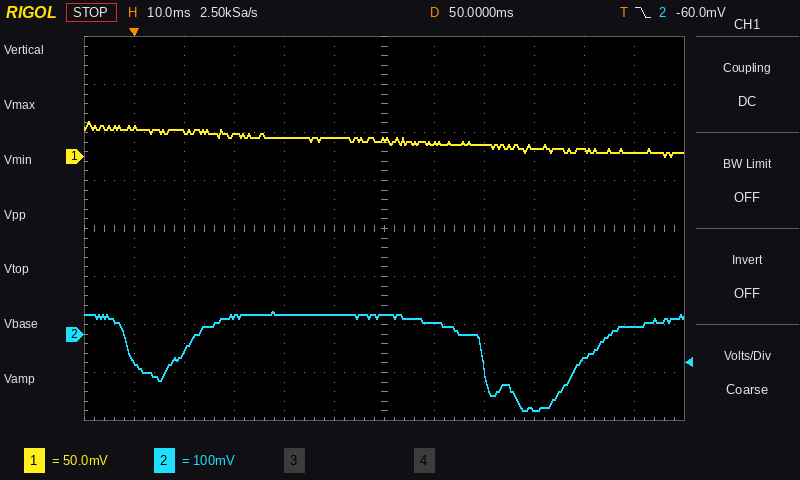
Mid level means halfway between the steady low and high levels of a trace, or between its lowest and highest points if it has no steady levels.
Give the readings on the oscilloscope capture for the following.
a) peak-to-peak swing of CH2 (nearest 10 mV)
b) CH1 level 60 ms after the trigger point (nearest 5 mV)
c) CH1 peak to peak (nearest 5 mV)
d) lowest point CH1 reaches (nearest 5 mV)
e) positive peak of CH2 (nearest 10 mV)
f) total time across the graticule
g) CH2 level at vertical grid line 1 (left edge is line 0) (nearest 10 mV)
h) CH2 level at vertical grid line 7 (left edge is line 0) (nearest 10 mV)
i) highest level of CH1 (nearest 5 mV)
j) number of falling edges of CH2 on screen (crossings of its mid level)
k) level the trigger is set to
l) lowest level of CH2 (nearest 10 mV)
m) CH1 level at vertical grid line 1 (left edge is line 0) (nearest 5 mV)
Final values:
210 mV
15 mV
35 mV
0 mV
50 mV
120 ms
-60 mV
20 mV
35 mV
2
-60.0 mV
-160 mV
30 mV
